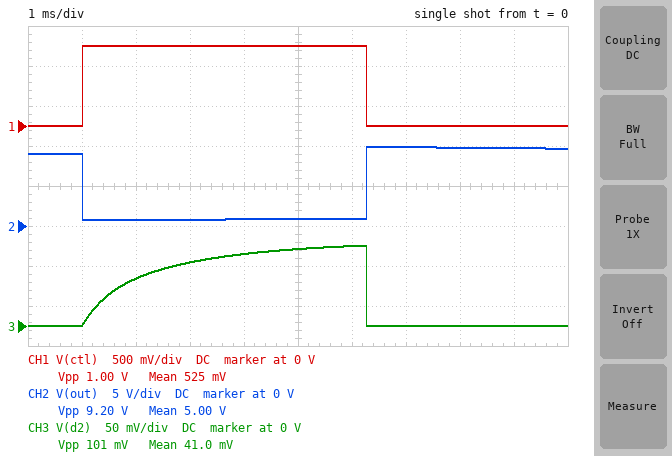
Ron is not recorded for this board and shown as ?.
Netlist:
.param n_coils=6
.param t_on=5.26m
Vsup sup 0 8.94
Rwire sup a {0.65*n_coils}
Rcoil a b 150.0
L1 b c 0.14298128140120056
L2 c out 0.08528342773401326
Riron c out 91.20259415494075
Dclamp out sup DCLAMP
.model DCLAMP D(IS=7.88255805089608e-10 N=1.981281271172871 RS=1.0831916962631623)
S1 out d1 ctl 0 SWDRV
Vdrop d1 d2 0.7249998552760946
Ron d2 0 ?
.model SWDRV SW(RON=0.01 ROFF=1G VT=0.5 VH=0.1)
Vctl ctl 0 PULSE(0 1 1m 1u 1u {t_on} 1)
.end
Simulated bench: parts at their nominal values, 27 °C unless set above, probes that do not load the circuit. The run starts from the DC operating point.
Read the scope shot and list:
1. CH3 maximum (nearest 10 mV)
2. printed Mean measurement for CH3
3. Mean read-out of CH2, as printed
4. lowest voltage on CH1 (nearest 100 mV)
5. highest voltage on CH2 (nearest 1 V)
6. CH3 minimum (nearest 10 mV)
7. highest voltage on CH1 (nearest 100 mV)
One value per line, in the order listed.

100 mV
41.0 mV
5.00 V
0 V
10 V
0 V
1.0 V
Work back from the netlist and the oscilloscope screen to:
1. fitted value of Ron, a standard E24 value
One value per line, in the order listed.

2 Ω
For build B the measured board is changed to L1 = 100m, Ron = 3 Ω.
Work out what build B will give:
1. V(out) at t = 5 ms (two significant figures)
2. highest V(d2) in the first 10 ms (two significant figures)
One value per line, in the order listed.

870 mV
150 mV
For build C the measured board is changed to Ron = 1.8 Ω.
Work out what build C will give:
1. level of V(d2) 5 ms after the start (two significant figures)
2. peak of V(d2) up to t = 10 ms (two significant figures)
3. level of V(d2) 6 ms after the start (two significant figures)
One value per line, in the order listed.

87 mV
91 mV
90 mV
